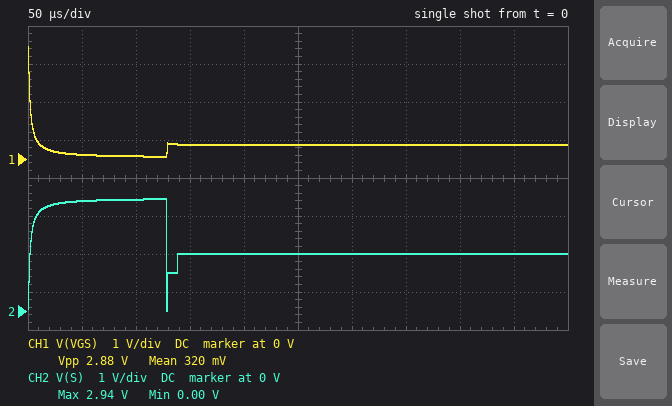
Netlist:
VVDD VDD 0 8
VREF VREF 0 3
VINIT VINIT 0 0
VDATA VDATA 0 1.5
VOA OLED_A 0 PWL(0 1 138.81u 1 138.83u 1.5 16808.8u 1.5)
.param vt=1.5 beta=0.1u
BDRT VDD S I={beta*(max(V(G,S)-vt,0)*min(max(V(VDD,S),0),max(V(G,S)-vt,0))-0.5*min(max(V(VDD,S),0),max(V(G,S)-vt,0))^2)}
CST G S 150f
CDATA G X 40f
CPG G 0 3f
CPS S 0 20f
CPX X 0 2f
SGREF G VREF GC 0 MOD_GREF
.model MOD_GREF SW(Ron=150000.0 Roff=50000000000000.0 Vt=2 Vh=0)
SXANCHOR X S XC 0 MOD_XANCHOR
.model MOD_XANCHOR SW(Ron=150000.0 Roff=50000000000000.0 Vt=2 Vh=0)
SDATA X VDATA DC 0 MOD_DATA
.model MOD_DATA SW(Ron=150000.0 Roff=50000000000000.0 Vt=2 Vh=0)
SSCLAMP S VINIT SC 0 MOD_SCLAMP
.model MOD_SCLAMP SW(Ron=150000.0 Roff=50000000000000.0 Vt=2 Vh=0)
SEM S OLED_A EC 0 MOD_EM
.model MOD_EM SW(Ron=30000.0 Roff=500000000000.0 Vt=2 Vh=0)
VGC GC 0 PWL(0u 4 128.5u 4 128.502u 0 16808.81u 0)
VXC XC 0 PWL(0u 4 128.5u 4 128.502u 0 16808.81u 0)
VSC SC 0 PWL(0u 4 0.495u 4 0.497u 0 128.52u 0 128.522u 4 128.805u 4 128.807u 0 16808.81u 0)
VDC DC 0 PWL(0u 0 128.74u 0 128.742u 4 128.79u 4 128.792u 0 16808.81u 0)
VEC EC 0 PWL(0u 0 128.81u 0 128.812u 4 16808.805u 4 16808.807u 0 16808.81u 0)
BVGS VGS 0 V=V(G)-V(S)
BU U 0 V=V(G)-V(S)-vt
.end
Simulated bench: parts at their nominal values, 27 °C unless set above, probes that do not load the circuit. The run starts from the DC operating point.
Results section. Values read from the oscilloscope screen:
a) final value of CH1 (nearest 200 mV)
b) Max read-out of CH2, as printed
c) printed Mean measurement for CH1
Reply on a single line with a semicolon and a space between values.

400 mV; 2.94 V; 320 mV
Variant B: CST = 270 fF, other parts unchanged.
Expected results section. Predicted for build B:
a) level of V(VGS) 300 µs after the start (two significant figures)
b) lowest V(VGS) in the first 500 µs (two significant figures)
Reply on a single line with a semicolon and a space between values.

270 mV; 77 mV
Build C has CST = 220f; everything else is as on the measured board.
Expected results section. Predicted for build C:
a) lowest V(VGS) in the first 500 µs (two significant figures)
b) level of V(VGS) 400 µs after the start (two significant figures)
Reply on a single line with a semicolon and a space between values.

70 mV; 300 mV
